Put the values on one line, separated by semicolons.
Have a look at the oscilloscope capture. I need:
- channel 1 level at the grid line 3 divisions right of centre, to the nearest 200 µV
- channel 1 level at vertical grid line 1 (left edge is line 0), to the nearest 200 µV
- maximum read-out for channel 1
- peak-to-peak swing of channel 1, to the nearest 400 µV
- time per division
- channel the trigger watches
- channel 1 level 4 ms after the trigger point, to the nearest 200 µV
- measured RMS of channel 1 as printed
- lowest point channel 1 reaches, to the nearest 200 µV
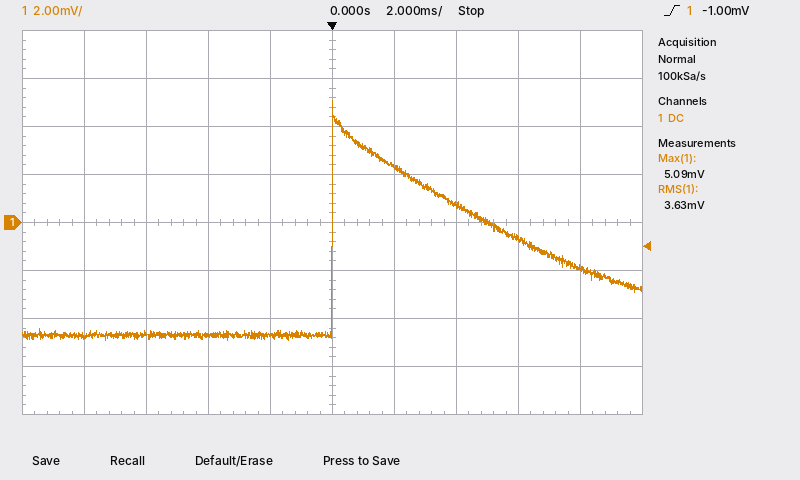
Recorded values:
-600 µV; -4.8 mV; 5.09 mV; 10.0 mV; 2 ms; channel 1; 800 µV; 3.63 mV; -5.0 mV
